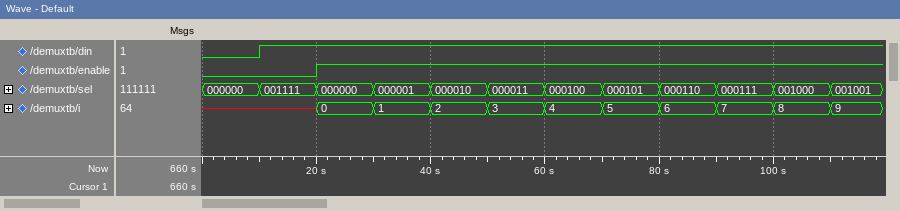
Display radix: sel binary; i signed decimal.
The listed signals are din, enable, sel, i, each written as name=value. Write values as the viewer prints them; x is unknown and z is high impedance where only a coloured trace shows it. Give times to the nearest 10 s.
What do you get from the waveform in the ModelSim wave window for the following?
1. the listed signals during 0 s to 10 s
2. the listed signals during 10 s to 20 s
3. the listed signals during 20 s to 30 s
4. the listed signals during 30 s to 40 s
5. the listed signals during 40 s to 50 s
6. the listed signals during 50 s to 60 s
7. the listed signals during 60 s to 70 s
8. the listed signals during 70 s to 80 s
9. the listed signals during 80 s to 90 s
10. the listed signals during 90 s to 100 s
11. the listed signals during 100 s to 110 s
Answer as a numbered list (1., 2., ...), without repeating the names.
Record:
1. din=0, enable=0, sel=000000, i=x
2. din=1, enable=0, sel=001111, i=x
3. din=1, enable=1, sel=000000, i=0
4. din=1, enable=1, sel=000001, i=1
5. din=1, enable=1, sel=000010, i=2
6. din=1, enable=1, sel=000011, i=3
7. din=1, enable=1, sel=000100, i=4
8. din=1, enable=1, sel=000101, i=5
9. din=1, enable=1, sel=000110, i=6
10. din=1, enable=1, sel=000111, i=7
11. din=1, enable=1, sel=001000, i=8
